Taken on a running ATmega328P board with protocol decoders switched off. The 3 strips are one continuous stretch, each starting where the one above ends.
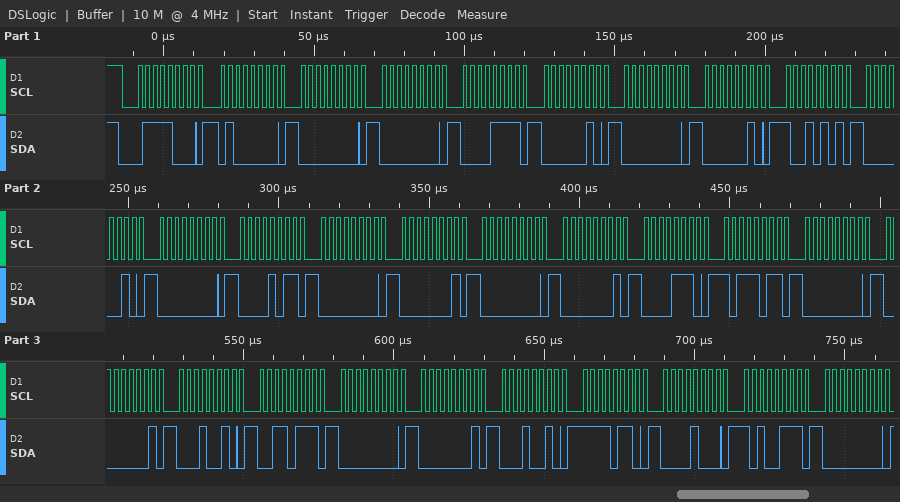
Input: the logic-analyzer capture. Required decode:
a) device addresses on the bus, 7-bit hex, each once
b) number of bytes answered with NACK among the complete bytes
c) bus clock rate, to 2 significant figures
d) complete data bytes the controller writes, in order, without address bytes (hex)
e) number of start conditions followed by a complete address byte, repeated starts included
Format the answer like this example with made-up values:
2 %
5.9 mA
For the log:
0x3C
0
400 kHz
40 00 00 0F 02 00 02 95 02 00 0B 00 01 00 01 0E BB 00 01 12 37 00 01 12 F6 08 A7 00
1
